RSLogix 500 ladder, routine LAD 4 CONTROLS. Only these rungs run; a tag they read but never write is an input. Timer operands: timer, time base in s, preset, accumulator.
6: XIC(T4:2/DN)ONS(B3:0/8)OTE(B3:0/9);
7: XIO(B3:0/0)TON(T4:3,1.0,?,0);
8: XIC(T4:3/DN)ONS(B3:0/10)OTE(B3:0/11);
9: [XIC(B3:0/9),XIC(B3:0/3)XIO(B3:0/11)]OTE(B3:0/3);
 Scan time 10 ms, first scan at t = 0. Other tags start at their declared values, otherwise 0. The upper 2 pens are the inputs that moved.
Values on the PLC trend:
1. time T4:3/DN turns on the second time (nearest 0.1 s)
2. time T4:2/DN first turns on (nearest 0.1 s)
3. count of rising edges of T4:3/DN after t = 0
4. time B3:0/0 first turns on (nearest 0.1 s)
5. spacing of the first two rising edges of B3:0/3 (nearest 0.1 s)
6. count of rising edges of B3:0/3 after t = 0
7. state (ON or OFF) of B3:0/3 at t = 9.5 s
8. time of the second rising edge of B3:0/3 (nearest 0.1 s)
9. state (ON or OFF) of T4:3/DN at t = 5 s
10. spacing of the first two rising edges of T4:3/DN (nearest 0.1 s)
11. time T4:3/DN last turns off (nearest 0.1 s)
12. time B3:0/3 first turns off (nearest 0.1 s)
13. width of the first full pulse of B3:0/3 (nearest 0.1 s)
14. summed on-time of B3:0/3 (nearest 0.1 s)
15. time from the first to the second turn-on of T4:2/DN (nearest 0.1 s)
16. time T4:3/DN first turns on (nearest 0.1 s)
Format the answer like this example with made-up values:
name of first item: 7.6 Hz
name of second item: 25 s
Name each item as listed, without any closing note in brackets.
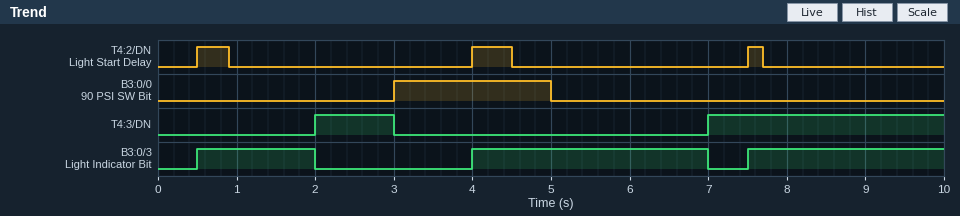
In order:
time T4:3/DN turns on the second time: 7.0 s
time T4:2/DN first turns on: 0.5 s
count of rising edges of T4:3/DN after t = 0: 2
time B3:0/0 first turns on: 3.0 s
spacing of the first two rising edges of B3:0/3: 3.5 s
count of rising edges of B3:0/3 after t = 0: 3
state (ON or OFF) of B3:0/3 at t = 9.5 s: ON
time of the second rising edge of B3:0/3: 4.0 s
state (ON or OFF) of T4:3/DN at t = 5 s: OFF
spacing of the first two rising edges of T4:3/DN: 5.0 s
time T4:3/DN last turns off: 3.0 s
time B3:0/3 first turns off: 2.0 s
width of the first full pulse of B3:0/3: 1.5 s
summed on-time of B3:0/3: 7.0 s
time from the first to the second turn-on of T4:2/DN: 3.5 s
time T4:3/DN first turns on: 2.0 s
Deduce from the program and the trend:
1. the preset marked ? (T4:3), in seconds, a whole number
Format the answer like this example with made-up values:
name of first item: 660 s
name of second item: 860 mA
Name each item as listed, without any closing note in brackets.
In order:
the preset marked ? (T4:3), in seconds, a whole number: 2 s
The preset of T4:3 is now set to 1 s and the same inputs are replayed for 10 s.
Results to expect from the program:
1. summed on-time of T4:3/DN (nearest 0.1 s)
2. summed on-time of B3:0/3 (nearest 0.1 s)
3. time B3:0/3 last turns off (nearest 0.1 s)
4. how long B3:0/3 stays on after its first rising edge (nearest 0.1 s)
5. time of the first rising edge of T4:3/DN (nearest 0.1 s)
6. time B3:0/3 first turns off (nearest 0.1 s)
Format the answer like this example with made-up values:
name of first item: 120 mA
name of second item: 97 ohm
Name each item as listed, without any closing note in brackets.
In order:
summed on-time of T4:3/DN: 6.0 s
summed on-time of B3:0/3: 5.0 s
time B3:0/3 last turns off: 6.0 s
how long B3:0/3 stays on after its first rising edge: 0.5 s
time of the first rising edge of T4:3/DN: 1.0 s
time B3:0/3 first turns off: 1.0 s
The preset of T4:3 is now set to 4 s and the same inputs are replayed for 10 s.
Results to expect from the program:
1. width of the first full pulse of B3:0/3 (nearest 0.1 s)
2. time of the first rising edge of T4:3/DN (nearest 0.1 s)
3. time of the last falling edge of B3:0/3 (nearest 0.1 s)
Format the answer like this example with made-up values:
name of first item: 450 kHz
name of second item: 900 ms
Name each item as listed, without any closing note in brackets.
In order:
width of the first full pulse of B3:0/3: 8.5 s
time of the first rising edge of T4:3/DN: 9.0 s
time of the last falling edge of B3:0/3: 9.0 s
